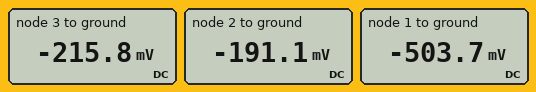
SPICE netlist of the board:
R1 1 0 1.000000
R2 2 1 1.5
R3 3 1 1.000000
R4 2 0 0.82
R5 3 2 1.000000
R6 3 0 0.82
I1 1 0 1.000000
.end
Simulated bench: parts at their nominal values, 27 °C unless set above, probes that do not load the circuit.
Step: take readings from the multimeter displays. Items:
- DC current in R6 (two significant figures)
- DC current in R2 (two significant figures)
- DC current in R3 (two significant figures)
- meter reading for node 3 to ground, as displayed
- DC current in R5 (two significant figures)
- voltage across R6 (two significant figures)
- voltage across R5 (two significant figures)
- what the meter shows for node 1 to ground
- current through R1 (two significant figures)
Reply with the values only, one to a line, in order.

260 mA
210 mA
290 mA
-215.8 mV
25 mA
220 mV
25 mV
-503.7 mV
500 mA
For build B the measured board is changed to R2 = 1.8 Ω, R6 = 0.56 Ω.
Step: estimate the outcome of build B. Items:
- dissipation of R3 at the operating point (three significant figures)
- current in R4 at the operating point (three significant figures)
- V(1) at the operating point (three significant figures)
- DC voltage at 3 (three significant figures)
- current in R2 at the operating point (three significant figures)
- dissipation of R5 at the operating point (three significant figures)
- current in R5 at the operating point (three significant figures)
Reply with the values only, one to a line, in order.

103 mW
197 mA
-494 mV
-173 mV
185 mA
140 µW
11.8 mA
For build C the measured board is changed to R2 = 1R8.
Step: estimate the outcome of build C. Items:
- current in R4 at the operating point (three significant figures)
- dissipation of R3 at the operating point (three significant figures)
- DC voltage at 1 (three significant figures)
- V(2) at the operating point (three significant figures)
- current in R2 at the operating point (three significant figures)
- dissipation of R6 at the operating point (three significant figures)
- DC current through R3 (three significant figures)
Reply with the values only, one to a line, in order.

221 mA
89.4 mW
-515 mV
-181 mV
186 mA
57.1 mW
299 mA
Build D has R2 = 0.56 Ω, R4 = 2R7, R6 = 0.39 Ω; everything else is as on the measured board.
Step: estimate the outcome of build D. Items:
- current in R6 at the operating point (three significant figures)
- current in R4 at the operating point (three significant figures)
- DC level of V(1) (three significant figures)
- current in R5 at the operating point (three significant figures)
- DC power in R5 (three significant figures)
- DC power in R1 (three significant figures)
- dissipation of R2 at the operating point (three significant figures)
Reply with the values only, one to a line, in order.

430 mA
115 mA
-455 mV
143 mA
20.4 mW
207 mW
37.2 mW
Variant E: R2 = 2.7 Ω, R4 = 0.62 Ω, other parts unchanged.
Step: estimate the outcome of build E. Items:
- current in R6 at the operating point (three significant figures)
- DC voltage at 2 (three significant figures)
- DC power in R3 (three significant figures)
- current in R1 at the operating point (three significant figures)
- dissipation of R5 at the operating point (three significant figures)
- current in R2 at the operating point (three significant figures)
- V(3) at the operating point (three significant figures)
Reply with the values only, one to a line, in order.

252 mA
-135 mV
105 mW
530 mA
5.12 mW
146 mA
-207 mV
